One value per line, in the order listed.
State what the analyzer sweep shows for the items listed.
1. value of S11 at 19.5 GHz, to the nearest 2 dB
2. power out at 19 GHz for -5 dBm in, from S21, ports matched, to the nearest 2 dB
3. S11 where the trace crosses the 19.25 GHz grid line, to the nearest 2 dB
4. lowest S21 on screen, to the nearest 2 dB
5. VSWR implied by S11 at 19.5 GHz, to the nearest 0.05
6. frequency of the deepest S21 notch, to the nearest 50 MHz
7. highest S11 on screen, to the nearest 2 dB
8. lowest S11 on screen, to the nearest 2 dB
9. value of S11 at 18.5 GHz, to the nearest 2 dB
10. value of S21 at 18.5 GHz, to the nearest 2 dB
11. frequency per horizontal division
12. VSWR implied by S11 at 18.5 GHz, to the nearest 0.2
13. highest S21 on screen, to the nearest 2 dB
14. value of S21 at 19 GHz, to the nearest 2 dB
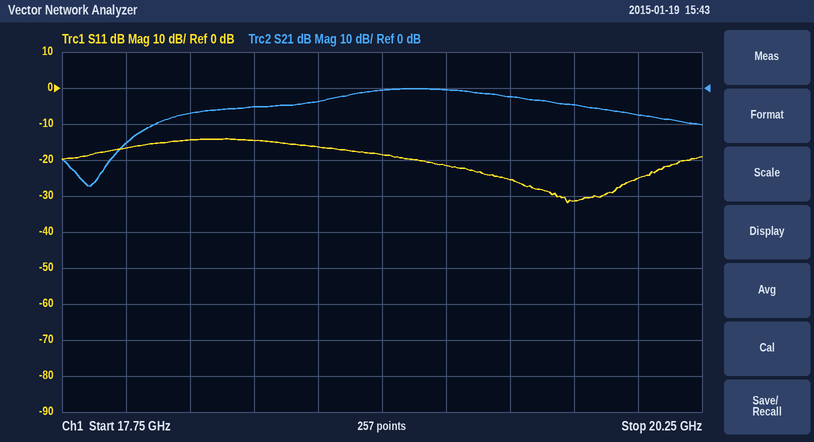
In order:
-26 dB
-6 dBm
-22 dB
-28 dB
1.10
17.85 GHz
-14 dB
-32 dB
-14 dB
-6 dB
250 MHz
1.4
0 dB
0 dB
